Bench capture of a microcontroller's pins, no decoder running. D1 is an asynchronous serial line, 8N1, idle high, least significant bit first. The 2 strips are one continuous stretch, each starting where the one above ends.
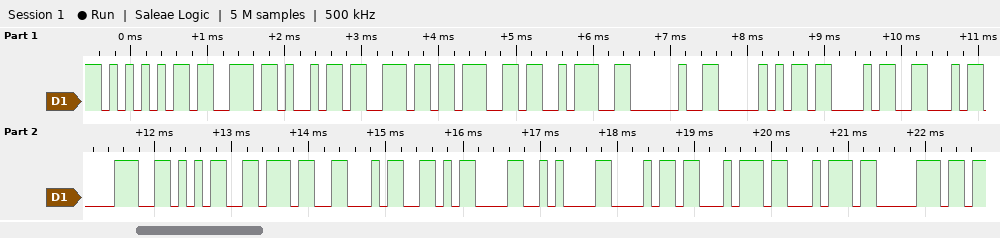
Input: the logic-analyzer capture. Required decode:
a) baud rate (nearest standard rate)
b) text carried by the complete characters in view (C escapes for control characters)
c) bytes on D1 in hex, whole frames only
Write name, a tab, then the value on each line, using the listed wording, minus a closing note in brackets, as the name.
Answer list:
baud rate	9600 baud
text carried by the complete characters in view	"Using: PCF8574\r\nhttp"
bytes on D1 in hex, whole frames only	55 73 69 6E 67 3A 20 50 43 46 38 35 37 34 0D 0A 68 74 74 70
